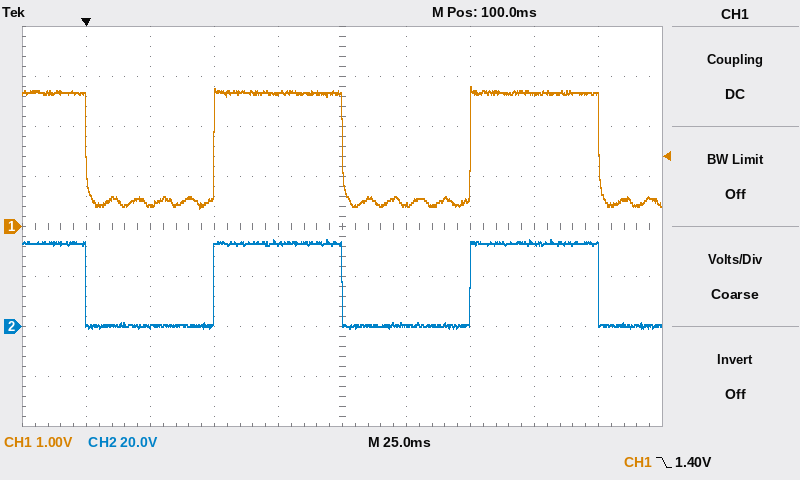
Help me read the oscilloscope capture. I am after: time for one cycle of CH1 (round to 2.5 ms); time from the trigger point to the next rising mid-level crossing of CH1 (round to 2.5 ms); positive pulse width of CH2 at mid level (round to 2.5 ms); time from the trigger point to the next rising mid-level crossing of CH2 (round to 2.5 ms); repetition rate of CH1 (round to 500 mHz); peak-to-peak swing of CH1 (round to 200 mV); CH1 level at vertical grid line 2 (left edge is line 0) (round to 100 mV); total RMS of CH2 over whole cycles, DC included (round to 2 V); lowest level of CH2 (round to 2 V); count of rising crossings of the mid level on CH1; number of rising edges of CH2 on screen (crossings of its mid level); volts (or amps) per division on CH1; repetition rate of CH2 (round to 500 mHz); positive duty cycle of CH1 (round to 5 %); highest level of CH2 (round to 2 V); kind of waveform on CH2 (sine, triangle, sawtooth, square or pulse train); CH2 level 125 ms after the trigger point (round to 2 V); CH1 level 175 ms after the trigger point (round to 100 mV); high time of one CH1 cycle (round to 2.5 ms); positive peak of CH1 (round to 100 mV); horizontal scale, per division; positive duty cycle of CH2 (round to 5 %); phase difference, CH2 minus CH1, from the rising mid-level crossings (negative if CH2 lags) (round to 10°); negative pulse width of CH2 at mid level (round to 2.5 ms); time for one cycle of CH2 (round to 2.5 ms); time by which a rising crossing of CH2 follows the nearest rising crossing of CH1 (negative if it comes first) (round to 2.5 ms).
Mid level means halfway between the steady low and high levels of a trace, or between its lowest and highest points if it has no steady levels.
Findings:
100.0 ms
50.0 ms
50.0 ms
50.0 ms
10.0 Hz
2.4 V
400 mV
24 V
0 V
2
2
1 V
10.0 Hz
50 %
34 V
square
0 V
2.7 V
50.0 ms
2.8 V
25 ms
50 %
0°
50.0 ms
100.0 ms
0.0 ms
